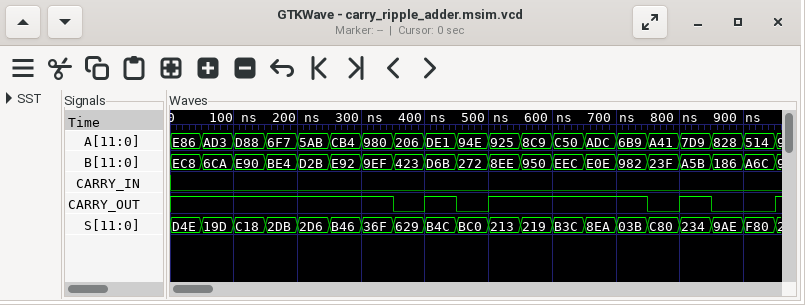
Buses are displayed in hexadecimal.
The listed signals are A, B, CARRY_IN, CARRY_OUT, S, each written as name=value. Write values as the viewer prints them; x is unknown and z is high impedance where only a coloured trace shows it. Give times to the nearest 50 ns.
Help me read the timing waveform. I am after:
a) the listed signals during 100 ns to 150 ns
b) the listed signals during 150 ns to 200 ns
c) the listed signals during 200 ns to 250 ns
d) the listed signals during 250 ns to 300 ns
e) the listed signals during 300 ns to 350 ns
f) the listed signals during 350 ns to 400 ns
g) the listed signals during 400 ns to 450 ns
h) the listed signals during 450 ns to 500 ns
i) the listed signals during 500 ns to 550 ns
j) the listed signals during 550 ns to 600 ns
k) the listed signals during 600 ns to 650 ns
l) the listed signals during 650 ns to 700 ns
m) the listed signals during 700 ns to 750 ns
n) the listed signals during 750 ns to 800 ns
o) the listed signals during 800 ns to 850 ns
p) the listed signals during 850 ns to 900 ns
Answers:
A=D88, B=E90, CARRY_IN=0, CARRY_OUT=1, S=C18
A=6F7, B=BE4, CARRY_IN=0, CARRY_OUT=1, S=2DB
A=5AB, B=D2B, CARRY_IN=0, CARRY_OUT=1, S=2D6
A=CB4, B=E92, CARRY_IN=0, CARRY_OUT=1, S=B46
A=980, B=9EF, CARRY_IN=0, CARRY_OUT=1, S=36F
A=206, B=423, CARRY_IN=0, CARRY_OUT=0, S=629
A=DE1, B=D6B, CARRY_IN=0, CARRY_OUT=1, S=B4C
A=94E, B=272, CARRY_IN=0, CARRY_OUT=0, S=BC0
A=925, B=8EE, CARRY_IN=0, CARRY_OUT=1, S=213
A=8C9, B=950, CARRY_IN=0, CARRY_OUT=1, S=219
A=C50, B=EEC, CARRY_IN=0, CARRY_OUT=1, S=B3C
A=ADC, B=E0E, CARRY_IN=0, CARRY_OUT=1, S=8EA
A=6B9, B=982, CARRY_IN=0, CARRY_OUT=1, S=03B
A=A41, B=23F, CARRY_IN=0, CARRY_OUT=0, S=C80
A=7D9, B=A5B, CARRY_IN=0, CARRY_OUT=1, S=234
A=828, B=186, CARRY_IN=0, CARRY_OUT=0, S=9AE
